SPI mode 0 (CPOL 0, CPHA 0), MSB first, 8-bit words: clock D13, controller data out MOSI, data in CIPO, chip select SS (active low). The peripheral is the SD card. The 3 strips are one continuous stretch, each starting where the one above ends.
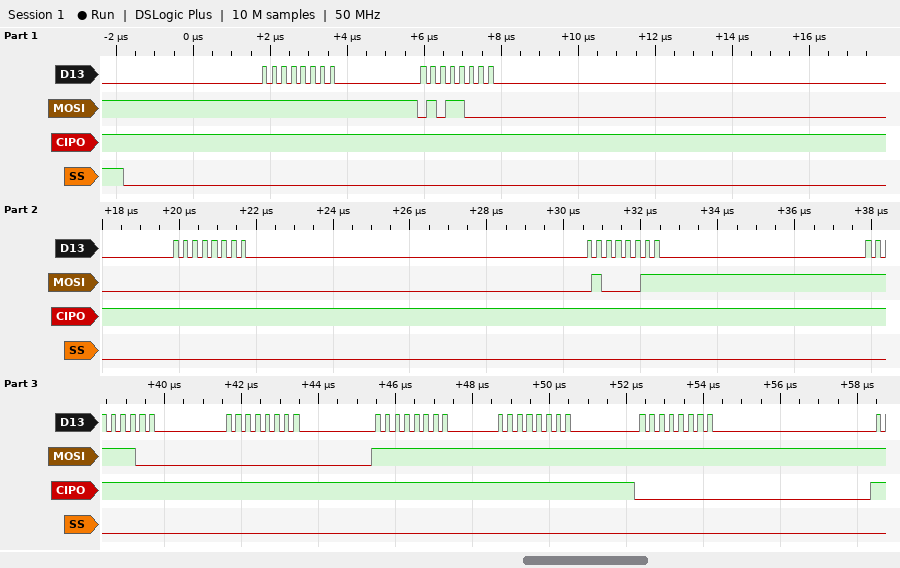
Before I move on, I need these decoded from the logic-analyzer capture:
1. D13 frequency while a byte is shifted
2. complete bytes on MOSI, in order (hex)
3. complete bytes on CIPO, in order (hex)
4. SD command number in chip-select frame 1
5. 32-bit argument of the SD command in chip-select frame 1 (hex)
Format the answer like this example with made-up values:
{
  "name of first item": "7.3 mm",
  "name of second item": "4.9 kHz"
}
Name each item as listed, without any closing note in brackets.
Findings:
{
  "D13 frequency while a byte is shifted": "4 MHz",
  "complete bytes on MOSI, in order": "0xFF 0x58 0x00 0x43 0xFC 0x00 0xFF 0xFF 0xFF",
  "complete bytes on CIPO, in order": "0xFF 0xFF 0xFF 0xFF 0xFF 0xFF 0xFF 0xFF 0x00",
  "SD command number in chip-select frame 1": "CMD24",
  "32-bit argument of the SD command in chip-select frame 1": "0x0043FC00"
}
